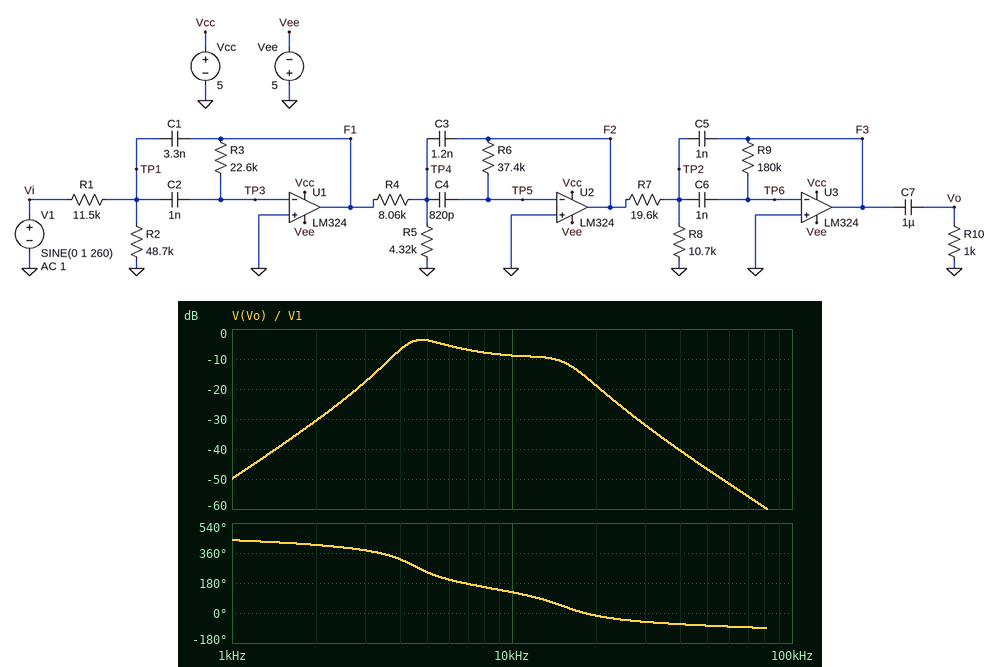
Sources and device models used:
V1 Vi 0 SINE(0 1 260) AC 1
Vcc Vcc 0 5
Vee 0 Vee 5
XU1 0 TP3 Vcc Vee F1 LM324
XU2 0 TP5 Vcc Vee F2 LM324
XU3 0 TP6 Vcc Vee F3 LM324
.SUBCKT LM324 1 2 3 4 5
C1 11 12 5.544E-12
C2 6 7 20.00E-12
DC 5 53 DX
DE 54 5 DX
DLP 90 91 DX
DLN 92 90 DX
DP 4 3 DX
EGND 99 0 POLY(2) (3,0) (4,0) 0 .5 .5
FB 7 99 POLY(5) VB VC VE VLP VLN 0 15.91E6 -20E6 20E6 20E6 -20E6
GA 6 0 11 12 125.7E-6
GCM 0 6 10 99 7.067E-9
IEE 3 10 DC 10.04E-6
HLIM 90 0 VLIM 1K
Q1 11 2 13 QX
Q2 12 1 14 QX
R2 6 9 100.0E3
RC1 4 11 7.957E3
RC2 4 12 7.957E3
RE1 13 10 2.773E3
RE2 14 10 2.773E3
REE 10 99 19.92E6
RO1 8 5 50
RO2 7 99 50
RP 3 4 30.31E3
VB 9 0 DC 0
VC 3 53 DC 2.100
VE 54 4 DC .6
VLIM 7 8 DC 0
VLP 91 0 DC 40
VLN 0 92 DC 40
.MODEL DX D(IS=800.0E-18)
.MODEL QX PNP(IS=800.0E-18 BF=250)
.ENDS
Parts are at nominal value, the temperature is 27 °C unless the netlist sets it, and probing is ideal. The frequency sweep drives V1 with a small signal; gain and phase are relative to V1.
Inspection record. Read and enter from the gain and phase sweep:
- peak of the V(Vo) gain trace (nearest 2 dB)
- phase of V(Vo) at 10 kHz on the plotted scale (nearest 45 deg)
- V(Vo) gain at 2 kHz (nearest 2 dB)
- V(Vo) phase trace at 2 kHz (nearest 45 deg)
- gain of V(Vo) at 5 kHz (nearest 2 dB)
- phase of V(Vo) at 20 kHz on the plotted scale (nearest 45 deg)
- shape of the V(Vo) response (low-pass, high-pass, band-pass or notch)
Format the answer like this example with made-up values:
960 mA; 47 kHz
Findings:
-4 dB; 135 deg; -30 dB; 405 deg; -4 dB; 0 deg; band-pass
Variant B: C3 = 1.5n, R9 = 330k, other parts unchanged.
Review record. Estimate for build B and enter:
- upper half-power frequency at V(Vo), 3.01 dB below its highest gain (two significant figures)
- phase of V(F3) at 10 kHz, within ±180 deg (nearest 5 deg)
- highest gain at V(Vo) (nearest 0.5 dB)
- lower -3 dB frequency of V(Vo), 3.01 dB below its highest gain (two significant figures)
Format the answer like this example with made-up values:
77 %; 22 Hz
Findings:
4.4 kHz; 110 deg; -3.0 dB; 3.0 kHz
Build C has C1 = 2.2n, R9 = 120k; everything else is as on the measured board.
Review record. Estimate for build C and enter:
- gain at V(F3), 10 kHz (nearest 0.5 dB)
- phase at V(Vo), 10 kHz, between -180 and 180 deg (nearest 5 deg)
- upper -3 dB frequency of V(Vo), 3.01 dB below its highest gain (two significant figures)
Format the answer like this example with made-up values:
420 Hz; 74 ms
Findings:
-4.5 dB; 145 deg; 13 kHz
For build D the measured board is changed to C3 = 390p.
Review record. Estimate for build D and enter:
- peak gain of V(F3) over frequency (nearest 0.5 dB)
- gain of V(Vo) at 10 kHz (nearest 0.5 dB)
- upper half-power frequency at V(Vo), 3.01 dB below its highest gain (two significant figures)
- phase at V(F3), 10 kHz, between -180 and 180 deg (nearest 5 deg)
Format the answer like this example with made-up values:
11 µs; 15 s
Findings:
-4.0 dB; -11.0 dB; 6.4 kHz; 140 deg
